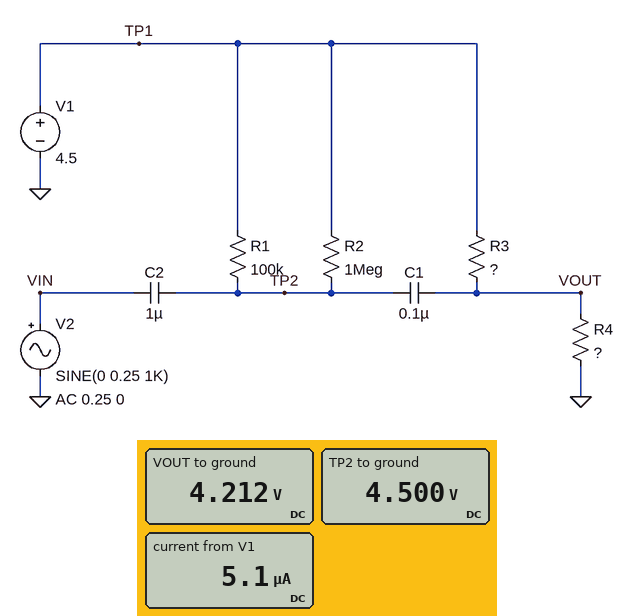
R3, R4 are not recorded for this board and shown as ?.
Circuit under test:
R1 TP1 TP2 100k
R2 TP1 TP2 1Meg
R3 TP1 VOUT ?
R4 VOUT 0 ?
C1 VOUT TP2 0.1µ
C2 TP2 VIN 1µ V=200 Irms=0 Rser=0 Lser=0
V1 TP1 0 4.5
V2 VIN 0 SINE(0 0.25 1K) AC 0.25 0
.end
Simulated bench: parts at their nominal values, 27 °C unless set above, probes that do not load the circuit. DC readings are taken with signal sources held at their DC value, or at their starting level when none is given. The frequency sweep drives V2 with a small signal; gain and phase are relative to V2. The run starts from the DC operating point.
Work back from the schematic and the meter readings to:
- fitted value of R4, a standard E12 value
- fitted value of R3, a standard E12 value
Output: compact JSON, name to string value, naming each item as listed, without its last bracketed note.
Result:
{"fitted value of R4, a standard E12 value": "820 kΩ", "fitted value of R3, a standard E12 value": "56 kΩ"}
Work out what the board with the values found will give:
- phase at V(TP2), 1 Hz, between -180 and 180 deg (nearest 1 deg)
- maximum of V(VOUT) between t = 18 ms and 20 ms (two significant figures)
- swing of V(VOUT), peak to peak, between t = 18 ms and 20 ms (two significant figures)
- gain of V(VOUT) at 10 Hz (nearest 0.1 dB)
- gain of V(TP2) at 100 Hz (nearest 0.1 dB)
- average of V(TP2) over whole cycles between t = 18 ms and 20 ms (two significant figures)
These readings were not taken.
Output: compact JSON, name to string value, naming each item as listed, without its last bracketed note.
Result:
{"phase at V(TP2), 1 Hz, between -180 and 180 deg": "58 deg", "maximum of V(VOUT) between t = 18 ms and 20 ms": "4.5 V", "swing of V(VOUT), peak to peak, between t = 18 ms and 20 ms": "500 mV", "gain of V(VOUT) at 10 Hz": "-11.0 dB", "gain of V(TP2) at 100 Hz": "-0.1 dB", "average of V(TP2) over whole cycles between t = 18 ms and 20 ms": "4.5 V"}
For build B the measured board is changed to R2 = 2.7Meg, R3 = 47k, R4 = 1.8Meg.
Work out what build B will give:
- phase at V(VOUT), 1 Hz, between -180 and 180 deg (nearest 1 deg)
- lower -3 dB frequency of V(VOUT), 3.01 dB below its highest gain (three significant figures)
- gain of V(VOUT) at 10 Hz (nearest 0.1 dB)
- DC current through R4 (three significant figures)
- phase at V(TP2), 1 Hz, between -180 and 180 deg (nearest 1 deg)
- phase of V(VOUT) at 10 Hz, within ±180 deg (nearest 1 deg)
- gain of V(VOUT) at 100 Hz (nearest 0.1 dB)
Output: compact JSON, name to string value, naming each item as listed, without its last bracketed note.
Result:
{"phase at V(VOUT), 1 Hz, between -180 and 180 deg": "145 deg", "lower -3 dB frequency of V(VOUT), 3.01 dB below its highest gain": "38.4 Hz", "gain of V(VOUT) at 10 Hz": "-12.1 dB", "DC current through R4": "2.44 µA", "phase at V(TP2), 1 Hz, between -180 and 180 deg": "56 deg", "phase of V(VOUT) at 10 Hz, within ±180 deg": "84 deg", "gain of V(VOUT) at 100 Hz": "-0.6 dB"}
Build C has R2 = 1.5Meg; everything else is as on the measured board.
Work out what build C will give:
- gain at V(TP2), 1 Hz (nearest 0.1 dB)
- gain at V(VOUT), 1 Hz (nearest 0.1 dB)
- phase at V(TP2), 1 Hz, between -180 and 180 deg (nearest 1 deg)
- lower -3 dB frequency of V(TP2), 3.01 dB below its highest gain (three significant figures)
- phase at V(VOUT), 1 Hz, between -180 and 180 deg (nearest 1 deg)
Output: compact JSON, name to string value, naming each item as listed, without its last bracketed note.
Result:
{"gain at V(TP2), 1 Hz": "-6.1 dB", "gain at V(VOUT), 1 Hz": "-35.8 dB", "phase at V(TP2), 1 Hz, between -180 and 180 deg": "57 deg", "lower -3 dB frequency of V(TP2), 3.01 dB below its highest gain": "1.92 Hz", "phase at V(VOUT), 1 Hz, between -180 and 180 deg": "145 deg"}
